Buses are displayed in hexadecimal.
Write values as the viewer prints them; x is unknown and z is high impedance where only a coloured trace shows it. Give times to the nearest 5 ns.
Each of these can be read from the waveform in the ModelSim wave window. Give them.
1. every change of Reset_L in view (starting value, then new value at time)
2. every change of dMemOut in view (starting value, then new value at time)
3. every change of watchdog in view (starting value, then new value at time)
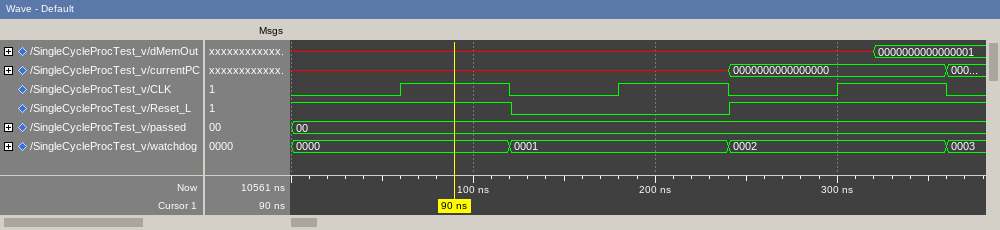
1, 0 at 120 ns, 1 at 240 ns
x, 0000000000000001 at 320 ns
0000, 0001 at 120 ns, 0002 at 240 ns, 0003 at 360 ns
